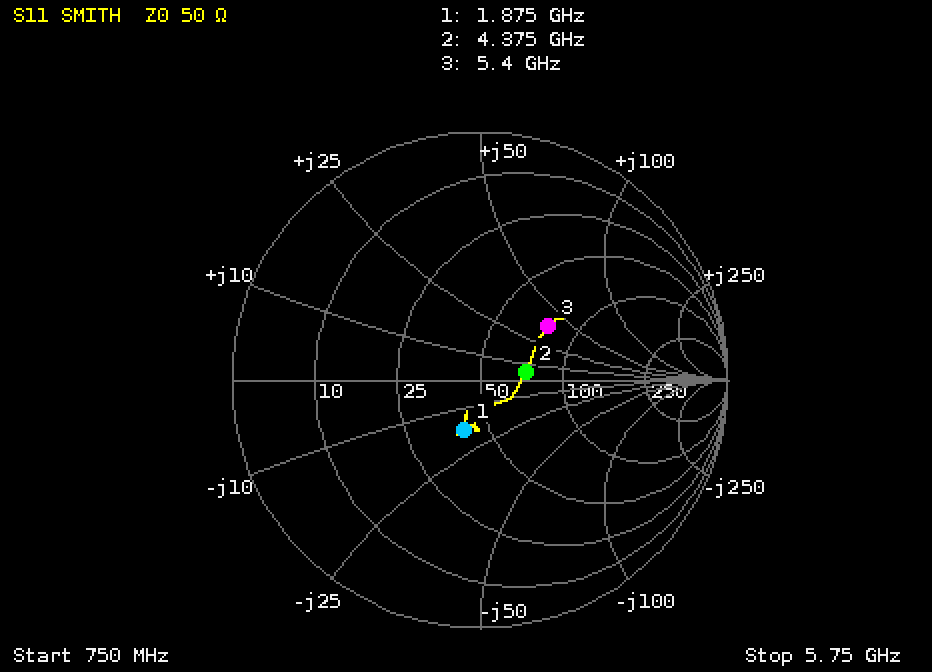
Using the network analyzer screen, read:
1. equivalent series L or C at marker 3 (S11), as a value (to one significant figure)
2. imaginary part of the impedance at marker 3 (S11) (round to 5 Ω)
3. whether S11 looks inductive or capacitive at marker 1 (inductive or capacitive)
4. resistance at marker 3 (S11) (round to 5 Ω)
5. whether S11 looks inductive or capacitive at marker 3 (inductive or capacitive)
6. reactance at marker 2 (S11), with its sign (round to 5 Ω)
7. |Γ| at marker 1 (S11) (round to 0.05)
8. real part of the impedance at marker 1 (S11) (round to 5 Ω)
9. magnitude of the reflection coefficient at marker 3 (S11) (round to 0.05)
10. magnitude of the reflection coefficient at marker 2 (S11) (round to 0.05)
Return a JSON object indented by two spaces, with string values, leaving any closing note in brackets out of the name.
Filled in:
{
  "equivalent series L or C at marker 3 (S11), as a value": "1 nH",
  "imaginary part of the impedance at marker 3 (S11)": "+40 Ω",
  "whether S11 looks inductive or capacitive at marker 1": "capacitive",
  "resistance at marker 3 (S11)": "75 Ω",
  "whether S11 looks inductive or capacitive at marker 3": "inductive",
  "reactance at marker 2 (S11), with its sign": "+5 Ω",
  "|Γ| at marker 1 (S11)": "0.20",
  "real part of the impedance at marker 1 (S11)": "40 Ω",
  "magnitude of the reflection coefficient at marker 3 (S11)": "0.35",
  "magnitude of the reflection coefficient at marker 2 (S11)": "0.20"
}
